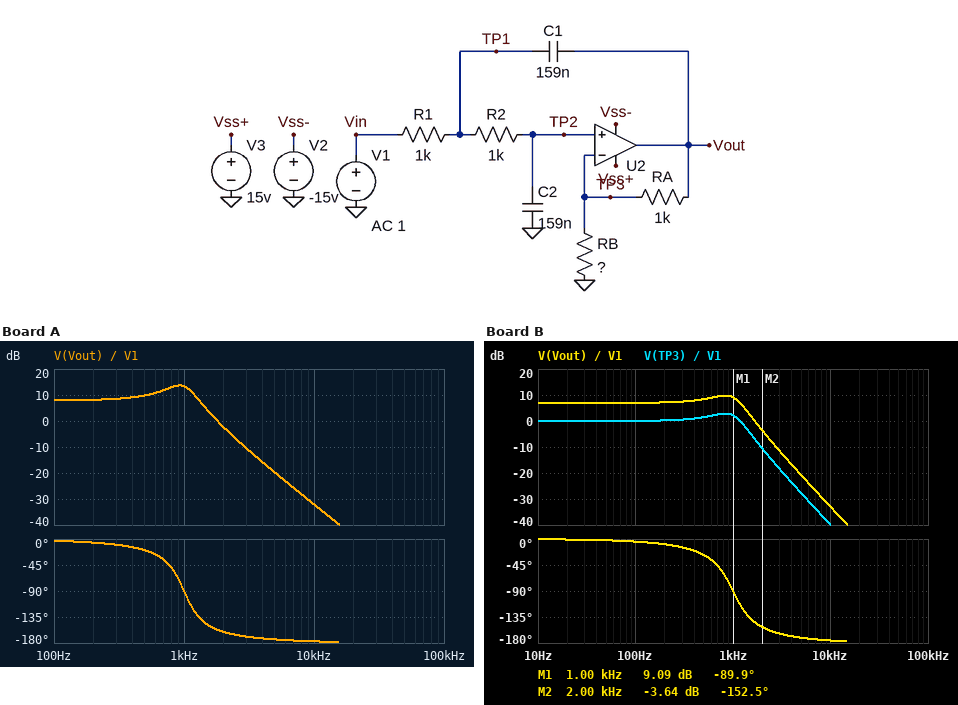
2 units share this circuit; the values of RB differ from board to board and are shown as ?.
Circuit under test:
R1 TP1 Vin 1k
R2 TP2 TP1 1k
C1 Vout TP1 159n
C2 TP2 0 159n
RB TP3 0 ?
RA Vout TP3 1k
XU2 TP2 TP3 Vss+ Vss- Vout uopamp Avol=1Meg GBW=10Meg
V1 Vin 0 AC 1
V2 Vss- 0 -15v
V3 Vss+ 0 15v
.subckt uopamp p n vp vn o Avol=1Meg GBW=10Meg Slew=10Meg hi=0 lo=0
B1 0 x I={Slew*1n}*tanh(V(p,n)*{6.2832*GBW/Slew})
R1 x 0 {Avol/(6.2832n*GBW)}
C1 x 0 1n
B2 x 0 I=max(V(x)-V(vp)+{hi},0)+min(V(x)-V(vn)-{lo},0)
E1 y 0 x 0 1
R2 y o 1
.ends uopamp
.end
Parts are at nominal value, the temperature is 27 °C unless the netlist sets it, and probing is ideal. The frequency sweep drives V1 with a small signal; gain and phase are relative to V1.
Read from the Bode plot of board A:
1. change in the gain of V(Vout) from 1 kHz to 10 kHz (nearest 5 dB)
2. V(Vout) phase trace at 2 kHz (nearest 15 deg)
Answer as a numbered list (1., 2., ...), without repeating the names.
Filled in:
1. -45 dB
2. -165 deg
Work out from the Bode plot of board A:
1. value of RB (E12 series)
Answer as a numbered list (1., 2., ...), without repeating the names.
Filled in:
1. 680 Ω
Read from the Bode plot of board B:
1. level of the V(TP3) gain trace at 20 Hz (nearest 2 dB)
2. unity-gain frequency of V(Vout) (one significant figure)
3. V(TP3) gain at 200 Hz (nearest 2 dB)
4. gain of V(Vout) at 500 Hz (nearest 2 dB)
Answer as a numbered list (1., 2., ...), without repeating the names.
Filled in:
1. 0 dB
2. 2 kHz
3. 0 dB
4. 8 dB
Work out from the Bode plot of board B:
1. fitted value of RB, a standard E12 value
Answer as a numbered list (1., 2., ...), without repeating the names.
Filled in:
1. 820 Ω
